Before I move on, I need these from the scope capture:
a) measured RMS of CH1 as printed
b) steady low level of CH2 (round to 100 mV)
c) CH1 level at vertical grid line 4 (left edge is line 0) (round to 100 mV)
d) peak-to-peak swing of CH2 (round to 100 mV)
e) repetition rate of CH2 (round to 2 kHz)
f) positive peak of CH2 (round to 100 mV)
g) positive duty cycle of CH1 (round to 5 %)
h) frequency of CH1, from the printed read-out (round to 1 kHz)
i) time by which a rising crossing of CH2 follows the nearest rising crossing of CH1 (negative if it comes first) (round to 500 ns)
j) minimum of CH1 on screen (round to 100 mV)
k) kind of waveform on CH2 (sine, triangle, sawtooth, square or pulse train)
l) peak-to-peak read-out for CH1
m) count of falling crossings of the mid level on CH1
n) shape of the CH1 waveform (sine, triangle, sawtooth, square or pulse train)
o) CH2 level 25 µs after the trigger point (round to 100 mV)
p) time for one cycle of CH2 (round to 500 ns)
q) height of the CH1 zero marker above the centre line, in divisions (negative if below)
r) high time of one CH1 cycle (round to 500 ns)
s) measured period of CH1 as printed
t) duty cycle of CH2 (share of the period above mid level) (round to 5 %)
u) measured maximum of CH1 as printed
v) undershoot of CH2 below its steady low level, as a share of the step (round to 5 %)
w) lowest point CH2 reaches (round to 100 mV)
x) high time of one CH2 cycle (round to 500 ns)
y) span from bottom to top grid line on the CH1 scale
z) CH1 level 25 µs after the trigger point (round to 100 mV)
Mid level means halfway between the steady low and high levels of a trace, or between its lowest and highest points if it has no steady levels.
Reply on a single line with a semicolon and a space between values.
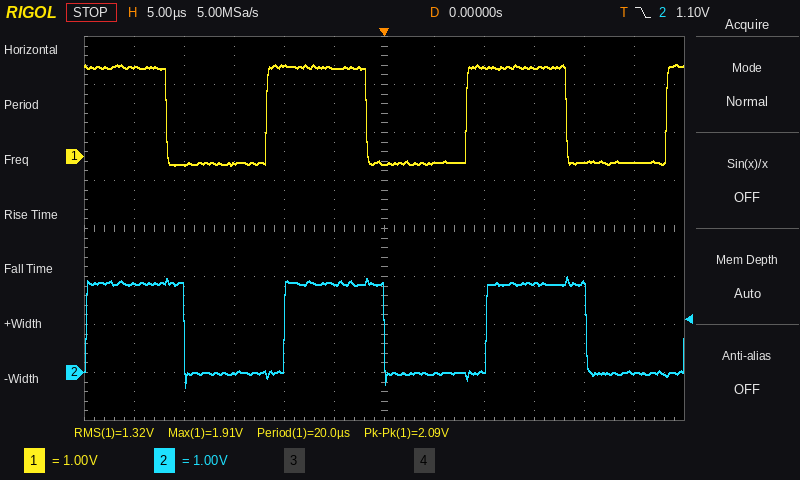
1.32 V; 0.0 V; 1.9 V; 2.3 V; 50 kHz; 2.0 V; 50 %; 50 kHz; +2.0 µs; -200 mV; square; 2.09 V; 3; square; 0.0 V; 20.0 µs; +1.5 div; 10.0 µs; 20.0 µs; 50 %; 1.91 V; 15 %; -300 mV; 10.0 µs; 8 V; -100 mV
